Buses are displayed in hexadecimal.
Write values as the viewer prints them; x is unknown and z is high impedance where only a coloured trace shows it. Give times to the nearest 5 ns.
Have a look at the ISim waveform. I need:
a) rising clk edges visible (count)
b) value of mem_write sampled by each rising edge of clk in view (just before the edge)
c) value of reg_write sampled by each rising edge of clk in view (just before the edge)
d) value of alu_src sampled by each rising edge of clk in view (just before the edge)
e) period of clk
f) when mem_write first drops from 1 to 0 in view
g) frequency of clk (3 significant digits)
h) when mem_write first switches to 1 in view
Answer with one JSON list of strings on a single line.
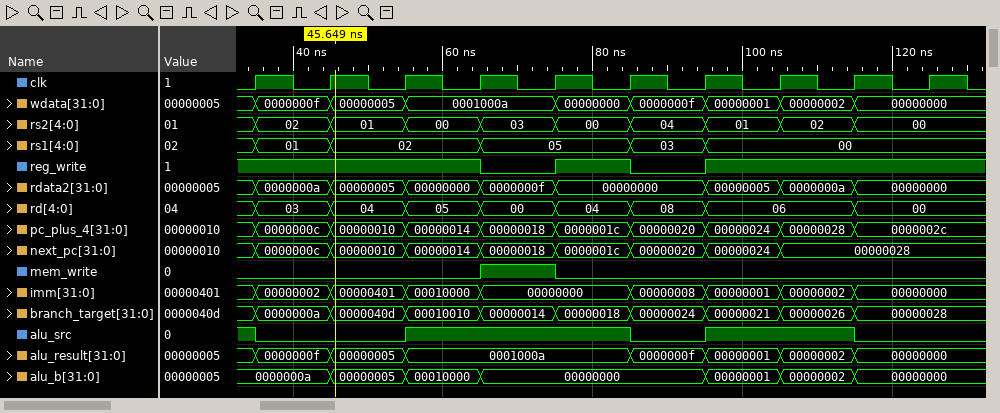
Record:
["10", "0 0 0 0 1 0 0 0 0 0", "1 1 1 1 0 1 0 1 1 1", "1 0 0 1 1 1 0 1 1 0", "10 ns", "75 ns", "100 MHz", "65 ns"]
